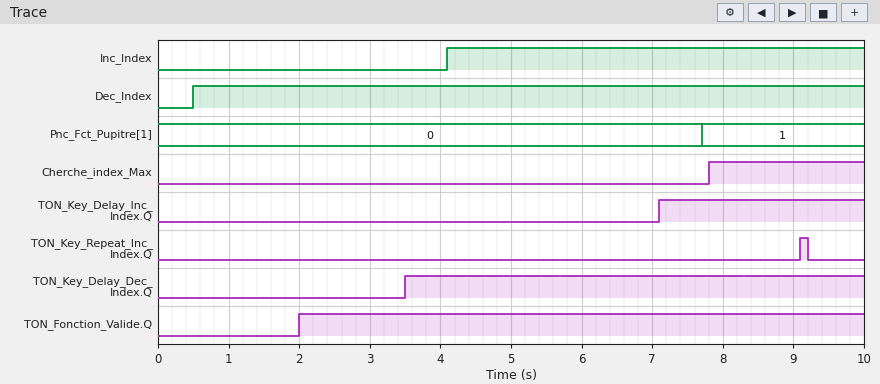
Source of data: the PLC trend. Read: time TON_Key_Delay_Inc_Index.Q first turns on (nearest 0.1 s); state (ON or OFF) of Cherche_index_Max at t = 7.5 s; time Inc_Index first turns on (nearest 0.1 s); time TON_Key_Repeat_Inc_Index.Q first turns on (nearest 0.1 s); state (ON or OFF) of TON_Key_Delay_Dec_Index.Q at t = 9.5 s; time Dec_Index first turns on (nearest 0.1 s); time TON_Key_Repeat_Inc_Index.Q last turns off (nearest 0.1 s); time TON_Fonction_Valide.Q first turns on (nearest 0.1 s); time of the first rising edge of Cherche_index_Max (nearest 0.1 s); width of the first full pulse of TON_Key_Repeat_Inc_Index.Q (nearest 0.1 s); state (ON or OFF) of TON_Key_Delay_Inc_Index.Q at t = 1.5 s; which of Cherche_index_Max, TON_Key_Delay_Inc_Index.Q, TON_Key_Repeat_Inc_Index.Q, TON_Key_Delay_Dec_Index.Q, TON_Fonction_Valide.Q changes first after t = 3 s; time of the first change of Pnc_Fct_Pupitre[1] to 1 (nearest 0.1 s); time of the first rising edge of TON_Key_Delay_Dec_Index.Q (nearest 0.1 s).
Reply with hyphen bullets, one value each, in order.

- 7.1 s
- OFF
- 4.1 s
- 9.1 s
- ON
- 0.5 s
- 9.2 s
- 2.0 s
- 7.8 s
- 0.1 s
- OFF
- TON_Key_Delay_Dec_Index.Q
- 7.7 s
- 3.5 s
